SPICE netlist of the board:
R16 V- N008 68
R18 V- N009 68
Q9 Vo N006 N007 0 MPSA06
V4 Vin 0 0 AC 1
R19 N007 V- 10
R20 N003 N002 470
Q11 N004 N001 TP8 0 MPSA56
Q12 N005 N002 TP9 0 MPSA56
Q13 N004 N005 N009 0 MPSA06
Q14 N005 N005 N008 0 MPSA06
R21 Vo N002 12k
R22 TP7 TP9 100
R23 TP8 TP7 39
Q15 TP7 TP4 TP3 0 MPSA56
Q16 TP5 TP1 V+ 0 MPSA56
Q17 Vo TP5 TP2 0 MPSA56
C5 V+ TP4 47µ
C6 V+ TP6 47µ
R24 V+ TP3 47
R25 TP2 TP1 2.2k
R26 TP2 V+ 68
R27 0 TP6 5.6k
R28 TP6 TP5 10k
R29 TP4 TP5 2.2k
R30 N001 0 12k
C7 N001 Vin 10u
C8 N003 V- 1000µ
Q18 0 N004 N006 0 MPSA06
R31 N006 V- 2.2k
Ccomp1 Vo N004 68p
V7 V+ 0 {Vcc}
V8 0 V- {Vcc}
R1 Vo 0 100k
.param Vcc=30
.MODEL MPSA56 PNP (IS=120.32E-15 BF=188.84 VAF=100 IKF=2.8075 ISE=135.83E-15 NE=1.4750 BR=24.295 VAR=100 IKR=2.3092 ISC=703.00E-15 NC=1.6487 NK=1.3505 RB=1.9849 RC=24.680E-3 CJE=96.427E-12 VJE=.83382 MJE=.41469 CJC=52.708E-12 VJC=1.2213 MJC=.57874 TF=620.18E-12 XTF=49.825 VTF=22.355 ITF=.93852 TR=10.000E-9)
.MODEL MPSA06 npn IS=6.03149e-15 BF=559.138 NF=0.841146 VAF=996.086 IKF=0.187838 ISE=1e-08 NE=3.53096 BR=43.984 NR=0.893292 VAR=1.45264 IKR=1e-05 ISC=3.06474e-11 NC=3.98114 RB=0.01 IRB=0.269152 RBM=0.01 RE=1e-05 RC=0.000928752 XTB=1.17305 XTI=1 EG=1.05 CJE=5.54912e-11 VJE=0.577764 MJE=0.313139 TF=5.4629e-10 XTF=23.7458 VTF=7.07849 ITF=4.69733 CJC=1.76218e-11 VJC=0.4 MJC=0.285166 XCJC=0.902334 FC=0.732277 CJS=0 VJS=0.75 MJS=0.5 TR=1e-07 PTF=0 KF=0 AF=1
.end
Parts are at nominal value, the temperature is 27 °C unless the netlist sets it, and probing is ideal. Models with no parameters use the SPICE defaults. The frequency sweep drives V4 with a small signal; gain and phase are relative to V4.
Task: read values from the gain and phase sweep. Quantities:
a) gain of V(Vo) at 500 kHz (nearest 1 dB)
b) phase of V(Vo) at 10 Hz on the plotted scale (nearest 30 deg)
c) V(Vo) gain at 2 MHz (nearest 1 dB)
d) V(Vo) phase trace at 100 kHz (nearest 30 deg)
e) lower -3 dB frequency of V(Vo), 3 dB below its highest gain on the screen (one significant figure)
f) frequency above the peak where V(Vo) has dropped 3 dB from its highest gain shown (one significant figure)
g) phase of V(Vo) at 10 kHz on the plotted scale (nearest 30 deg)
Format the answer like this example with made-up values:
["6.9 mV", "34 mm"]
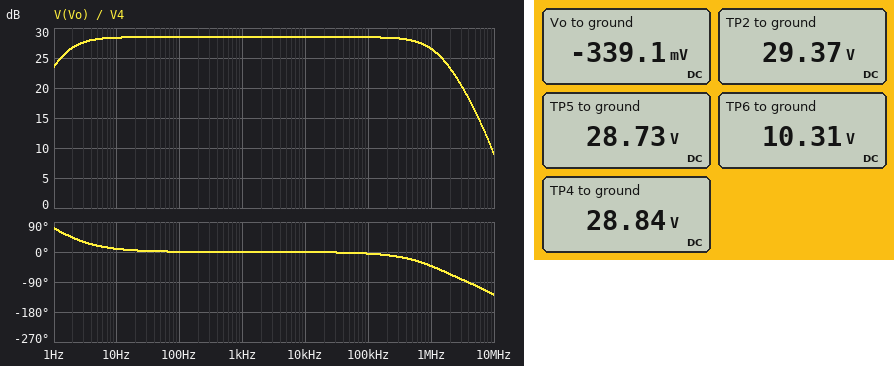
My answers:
["28 dB", "0 deg", "23 dB", "0 deg", "1 Hz", "1 MHz", "0 deg"]
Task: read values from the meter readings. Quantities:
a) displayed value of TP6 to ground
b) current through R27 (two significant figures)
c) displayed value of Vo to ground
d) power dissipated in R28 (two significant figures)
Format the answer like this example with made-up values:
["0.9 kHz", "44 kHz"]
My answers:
["10.31 V", "1.8 mA", "-339.1 mV", "34 mW"]
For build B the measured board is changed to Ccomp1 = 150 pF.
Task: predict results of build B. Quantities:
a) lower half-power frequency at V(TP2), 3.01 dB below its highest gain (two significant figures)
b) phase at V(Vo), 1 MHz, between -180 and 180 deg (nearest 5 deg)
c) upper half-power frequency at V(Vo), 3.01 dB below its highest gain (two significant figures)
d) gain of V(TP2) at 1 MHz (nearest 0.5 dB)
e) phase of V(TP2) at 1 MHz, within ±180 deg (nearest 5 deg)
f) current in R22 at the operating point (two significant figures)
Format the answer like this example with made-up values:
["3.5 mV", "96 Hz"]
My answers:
["1.4 MHz", "-65 deg", "560 kHz", "-29.5 dB", "50 deg", "5.5 mA"]
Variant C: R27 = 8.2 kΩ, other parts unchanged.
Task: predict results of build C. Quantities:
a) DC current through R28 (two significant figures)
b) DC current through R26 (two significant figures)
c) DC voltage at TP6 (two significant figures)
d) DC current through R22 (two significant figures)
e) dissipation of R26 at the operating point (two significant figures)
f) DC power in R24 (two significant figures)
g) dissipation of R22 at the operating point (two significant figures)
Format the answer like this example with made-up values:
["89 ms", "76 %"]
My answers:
["1.6 mA", "9.1 mA", "13 V", "5.4 mA", "5.7 mW", "5.5 mW", "2.9 mW"]
